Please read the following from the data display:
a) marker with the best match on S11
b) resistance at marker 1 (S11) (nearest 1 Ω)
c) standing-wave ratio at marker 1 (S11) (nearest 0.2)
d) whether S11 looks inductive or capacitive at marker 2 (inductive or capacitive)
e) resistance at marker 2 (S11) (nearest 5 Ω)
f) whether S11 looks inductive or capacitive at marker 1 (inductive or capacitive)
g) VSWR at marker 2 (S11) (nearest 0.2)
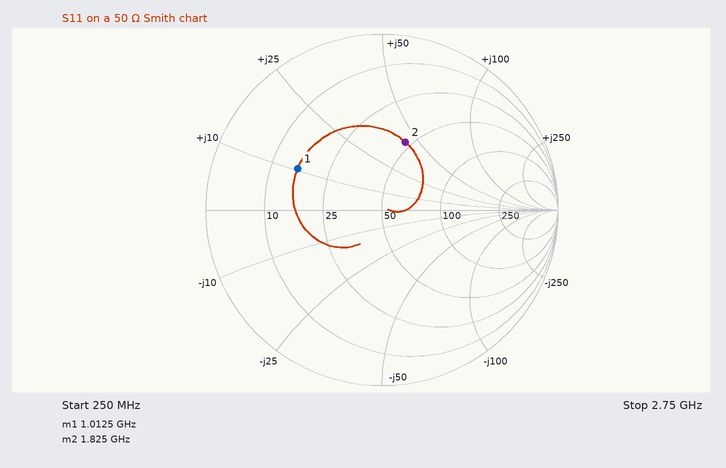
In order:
marker 2
16 Ω
3.2
inductive
45 Ω
inductive
2.4
